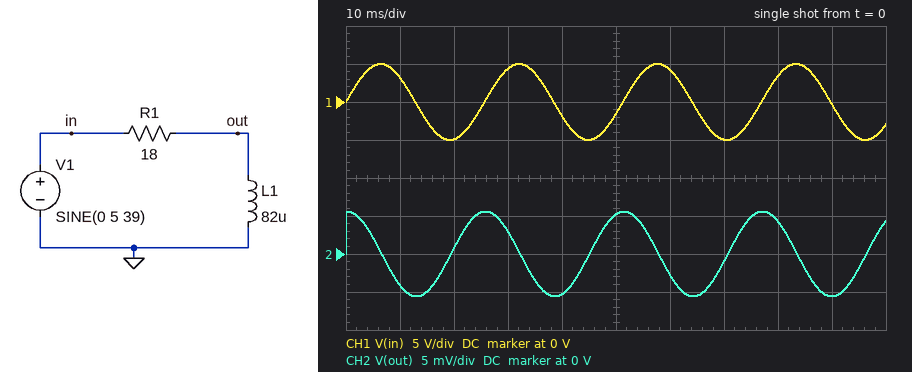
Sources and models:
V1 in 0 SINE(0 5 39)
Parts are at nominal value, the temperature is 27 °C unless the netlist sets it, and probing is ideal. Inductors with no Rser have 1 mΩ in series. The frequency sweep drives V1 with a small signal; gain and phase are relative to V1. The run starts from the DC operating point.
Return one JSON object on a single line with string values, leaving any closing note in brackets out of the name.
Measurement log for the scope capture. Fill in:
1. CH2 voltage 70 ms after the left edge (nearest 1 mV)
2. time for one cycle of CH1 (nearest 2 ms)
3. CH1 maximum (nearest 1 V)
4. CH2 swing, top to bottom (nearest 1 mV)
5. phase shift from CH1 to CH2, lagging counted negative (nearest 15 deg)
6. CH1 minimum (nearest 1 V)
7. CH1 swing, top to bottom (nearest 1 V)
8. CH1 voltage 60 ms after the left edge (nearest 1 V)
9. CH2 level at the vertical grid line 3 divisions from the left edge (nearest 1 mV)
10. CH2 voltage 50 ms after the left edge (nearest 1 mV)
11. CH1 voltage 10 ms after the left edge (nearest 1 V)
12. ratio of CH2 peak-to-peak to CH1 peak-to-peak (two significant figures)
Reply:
{"CH2 voltage 70 ms after the left edge": "-1 mV", "time for one cycle of CH1": "26 ms", "CH1 maximum": "5 V", "CH2 swing, top to bottom": "11 mV", "phase shift from CH1 to CH2, lagging counted negative": "90 deg", "CH1 minimum": "-5 V", "CH1 swing, top to bottom": "10 V", "CH1 voltage 60 ms after the left edge": "4 V", "CH2 level at the vertical grid line 3 divisions from the left edge": "3 mV", "CH2 voltage 50 ms after the left edge": "5 mV", "CH1 voltage 10 ms after the left edge": "3 V", "ratio of CH2 peak-to-peak to CH1 peak-to-peak": "0.0011"}
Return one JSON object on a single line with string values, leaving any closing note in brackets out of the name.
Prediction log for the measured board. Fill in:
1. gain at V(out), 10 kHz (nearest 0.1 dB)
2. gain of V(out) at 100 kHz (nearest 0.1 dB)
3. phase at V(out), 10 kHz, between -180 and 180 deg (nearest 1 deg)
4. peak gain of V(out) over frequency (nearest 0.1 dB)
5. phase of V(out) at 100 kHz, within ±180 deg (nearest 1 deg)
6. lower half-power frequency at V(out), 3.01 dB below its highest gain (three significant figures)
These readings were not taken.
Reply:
{"gain at V(out), 10 kHz": "-11.2 dB", "gain of V(out) at 100 kHz": "-0.5 dB", "phase at V(out), 10 kHz, between -180 and 180 deg": "74 deg", "peak gain of V(out) over frequency": "0 dB", "phase of V(out) at 100 kHz, within ±180 deg": "19 deg", "lower half-power frequency at V(out), 3.01 dB below its highest gain": "34.9 kHz"}
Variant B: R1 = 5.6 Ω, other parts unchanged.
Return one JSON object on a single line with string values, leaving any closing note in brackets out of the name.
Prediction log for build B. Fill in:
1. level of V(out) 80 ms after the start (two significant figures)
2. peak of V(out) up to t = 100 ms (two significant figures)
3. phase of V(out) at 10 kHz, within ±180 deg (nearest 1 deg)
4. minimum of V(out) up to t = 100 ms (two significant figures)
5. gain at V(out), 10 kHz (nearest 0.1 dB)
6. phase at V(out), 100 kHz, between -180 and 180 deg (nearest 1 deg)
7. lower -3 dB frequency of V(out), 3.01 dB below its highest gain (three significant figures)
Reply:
{"level of V(out) 80 ms after the start": "14 mV", "peak of V(out) up to t = 100 ms": "18 mV", "phase of V(out) at 10 kHz, within ±180 deg": "47 deg", "minimum of V(out) up to t = 100 ms": "-18 mV", "gain at V(out), 10 kHz": "-3.4 dB", "phase at V(out), 100 kHz, between -180 and 180 deg": "6 deg", "lower -3 dB frequency of V(out), 3.01 dB below its highest gain": "10.9 kHz"}
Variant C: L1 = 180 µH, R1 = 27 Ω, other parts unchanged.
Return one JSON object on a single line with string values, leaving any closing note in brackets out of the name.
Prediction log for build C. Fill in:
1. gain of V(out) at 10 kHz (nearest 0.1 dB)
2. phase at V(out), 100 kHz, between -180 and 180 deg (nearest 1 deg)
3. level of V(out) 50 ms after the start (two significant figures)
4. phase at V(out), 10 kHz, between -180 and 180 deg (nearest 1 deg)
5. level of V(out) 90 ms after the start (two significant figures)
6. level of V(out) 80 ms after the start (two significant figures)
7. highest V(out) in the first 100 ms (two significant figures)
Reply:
{"gain of V(out) at 10 kHz": "-8.3 dB", "phase at V(out), 100 kHz, between -180 and 180 deg": "13 deg", "level of V(out) 50 ms after the start": "7.7 mV", "phase at V(out), 10 kHz, between -180 and 180 deg": "67 deg", "level of V(out) 90 ms after the start": "-8.2 mV", "level of V(out) 80 ms after the start": "6.1 mV", "highest V(out) in the first 100 ms": "8.2 mV"}
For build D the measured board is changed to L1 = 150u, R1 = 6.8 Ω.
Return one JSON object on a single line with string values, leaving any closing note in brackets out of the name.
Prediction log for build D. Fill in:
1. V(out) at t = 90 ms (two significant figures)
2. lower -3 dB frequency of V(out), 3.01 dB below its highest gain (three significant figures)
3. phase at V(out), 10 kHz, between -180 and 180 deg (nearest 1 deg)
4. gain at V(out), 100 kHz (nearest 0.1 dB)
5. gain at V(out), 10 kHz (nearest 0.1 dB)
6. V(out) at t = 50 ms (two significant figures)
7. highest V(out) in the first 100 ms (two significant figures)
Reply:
{"V(out) at t = 90 ms": "-27 mV", "lower -3 dB frequency of V(out), 3.01 dB below its highest gain": "7.22 kHz", "phase at V(out), 10 kHz, between -180 and 180 deg": "36 deg", "gain at V(out), 100 kHz": "0 dB", "gain at V(out), 10 kHz": "-1.8 dB", "V(out) at t = 50 ms": "25 mV", "highest V(out) in the first 100 ms": "27 mV"}
